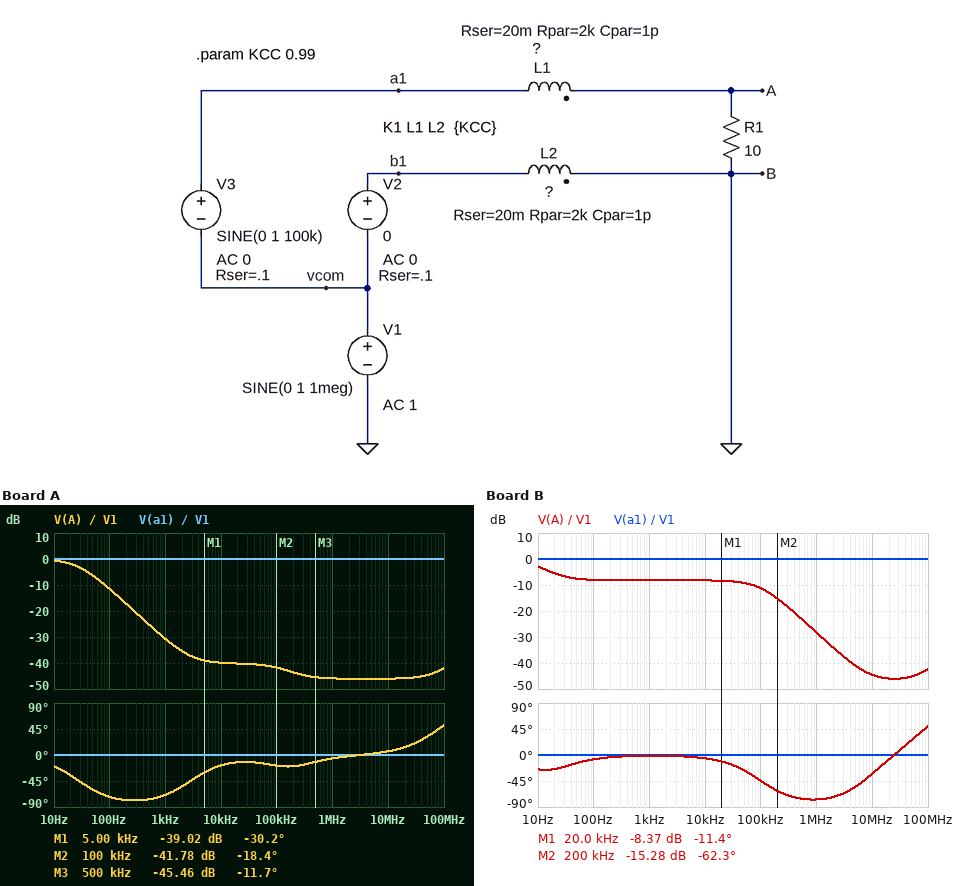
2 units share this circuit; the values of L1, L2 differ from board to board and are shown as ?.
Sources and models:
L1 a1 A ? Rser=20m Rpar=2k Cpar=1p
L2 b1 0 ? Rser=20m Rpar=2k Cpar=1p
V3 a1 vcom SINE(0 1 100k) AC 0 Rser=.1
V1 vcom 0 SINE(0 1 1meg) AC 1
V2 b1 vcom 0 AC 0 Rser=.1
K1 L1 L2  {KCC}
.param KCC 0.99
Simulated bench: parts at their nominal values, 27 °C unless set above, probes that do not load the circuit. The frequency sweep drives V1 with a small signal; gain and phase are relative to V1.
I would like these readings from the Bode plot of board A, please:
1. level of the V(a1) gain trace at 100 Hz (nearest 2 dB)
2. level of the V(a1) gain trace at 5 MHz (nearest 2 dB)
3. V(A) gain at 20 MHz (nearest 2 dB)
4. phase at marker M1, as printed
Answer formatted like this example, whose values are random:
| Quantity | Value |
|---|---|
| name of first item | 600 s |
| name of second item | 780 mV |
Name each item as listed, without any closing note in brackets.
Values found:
| Quantity | Value |
|---|---|
| level of the V(a1) gain trace at 100 Hz | 0 dB |
| level of the V(a1) gain trace at 5 MHz | 0 dB |
| V(A) gain at 20 MHz | -46 dB |
| phase at marker M1, as printed | -30.2 deg |
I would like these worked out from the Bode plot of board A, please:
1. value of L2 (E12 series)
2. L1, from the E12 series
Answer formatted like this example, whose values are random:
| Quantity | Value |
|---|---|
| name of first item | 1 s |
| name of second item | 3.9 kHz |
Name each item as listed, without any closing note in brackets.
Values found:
| Quantity | Value |
|---|---|
| value of L2 | 680 µH |
| L1, from the E12 series | 680 µH |
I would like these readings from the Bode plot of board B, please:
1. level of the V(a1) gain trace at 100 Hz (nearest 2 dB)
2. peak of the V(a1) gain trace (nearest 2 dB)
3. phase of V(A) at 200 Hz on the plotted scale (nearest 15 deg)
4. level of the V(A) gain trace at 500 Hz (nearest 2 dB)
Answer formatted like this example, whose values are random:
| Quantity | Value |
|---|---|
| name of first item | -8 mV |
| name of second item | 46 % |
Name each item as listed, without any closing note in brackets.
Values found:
| Quantity | Value |
|---|---|
| level of the V(a1) gain trace at 100 Hz | 0 dB |
| peak of the V(a1) gain trace | 0 dB |
| phase of V(A) at 200 Hz on the plotted scale | 0 deg |
| level of the V(A) gain trace at 500 Hz | -8 dB |
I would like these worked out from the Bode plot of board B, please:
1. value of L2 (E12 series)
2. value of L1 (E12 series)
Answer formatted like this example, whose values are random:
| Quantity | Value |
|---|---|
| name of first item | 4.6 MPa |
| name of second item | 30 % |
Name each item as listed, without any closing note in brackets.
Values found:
| Quantity | Value |
|---|---|
| value of L2 | 2.2 mH |
| value of L1 | 820 µH |
